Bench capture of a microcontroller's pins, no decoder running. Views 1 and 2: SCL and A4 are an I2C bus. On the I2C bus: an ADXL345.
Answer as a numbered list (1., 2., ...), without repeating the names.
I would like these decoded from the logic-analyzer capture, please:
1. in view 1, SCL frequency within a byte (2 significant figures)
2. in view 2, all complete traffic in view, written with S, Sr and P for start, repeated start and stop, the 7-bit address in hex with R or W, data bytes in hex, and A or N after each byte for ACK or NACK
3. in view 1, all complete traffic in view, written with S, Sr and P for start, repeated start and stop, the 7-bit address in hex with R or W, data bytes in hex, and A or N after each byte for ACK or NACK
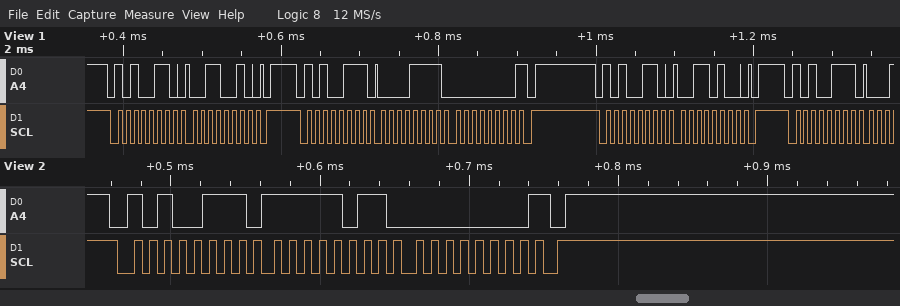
1. 100 kHz
2. S 53R A FB A 00 N P
3. S 53W A 32 A P S 53R A 0F A 00 N P S 53W A 34 A P S 53R A
